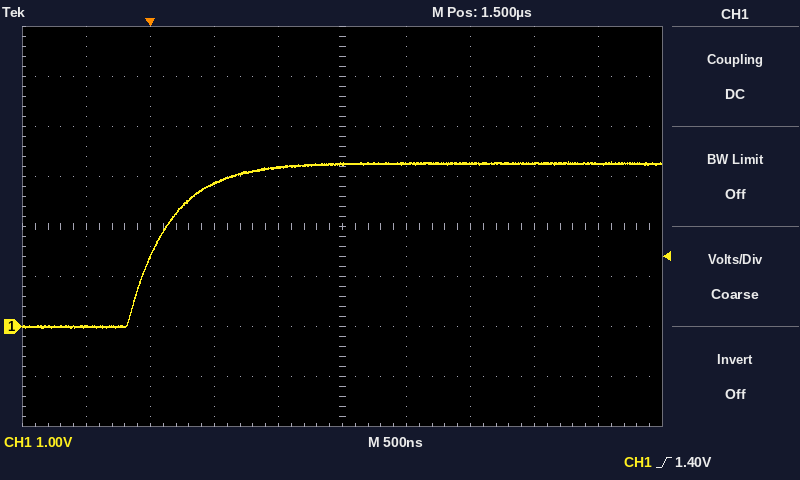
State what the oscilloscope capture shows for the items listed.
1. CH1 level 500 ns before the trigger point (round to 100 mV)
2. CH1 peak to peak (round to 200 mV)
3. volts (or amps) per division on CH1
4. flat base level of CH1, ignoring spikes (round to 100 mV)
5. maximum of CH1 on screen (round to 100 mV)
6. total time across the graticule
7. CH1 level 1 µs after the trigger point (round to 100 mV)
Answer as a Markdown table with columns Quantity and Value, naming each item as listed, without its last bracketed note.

| Quantity | Value |
|---|---|
| CH1 level 500 ns before the trigger point | 0.0 V |
| CH1 peak to peak | 3.4 V |
| volts (or amps) per division on CH1 | 1 V |
| flat base level of CH1, ignoring spikes | 0.0 V |
| maximum of CH1 on screen | 3.3 V |
| total time across the graticule | 5 µs |
| CH1 level 1 µs after the trigger point | 3.2 V |
